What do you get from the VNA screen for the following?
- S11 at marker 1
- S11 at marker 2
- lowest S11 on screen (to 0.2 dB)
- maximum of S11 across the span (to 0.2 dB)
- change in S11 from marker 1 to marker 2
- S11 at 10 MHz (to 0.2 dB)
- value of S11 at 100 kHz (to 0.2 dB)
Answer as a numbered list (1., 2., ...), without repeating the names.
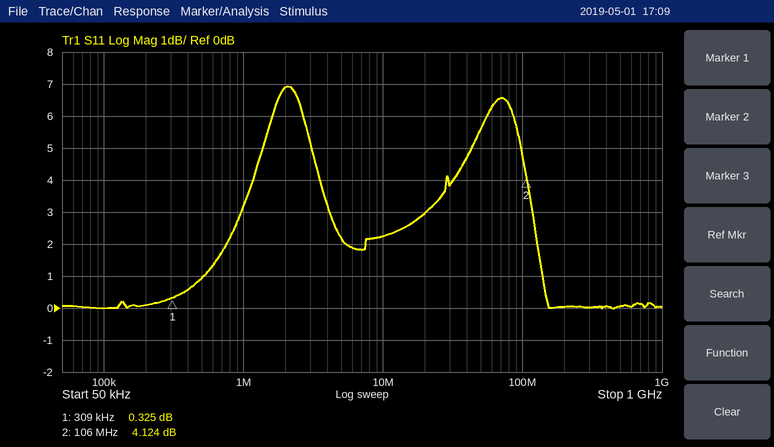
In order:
1. 0.325 dB
2. 4.124 dB
3. 0.0 dB
4. 7.0 dB
5. 3.799 dB
6. 2.2 dB
7. 0.0 dB
